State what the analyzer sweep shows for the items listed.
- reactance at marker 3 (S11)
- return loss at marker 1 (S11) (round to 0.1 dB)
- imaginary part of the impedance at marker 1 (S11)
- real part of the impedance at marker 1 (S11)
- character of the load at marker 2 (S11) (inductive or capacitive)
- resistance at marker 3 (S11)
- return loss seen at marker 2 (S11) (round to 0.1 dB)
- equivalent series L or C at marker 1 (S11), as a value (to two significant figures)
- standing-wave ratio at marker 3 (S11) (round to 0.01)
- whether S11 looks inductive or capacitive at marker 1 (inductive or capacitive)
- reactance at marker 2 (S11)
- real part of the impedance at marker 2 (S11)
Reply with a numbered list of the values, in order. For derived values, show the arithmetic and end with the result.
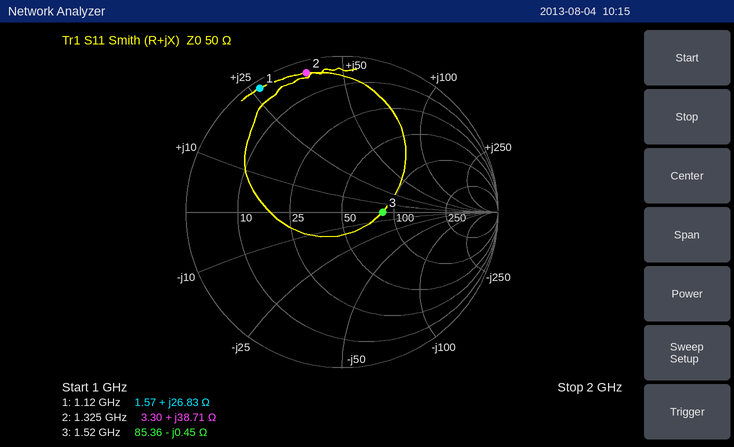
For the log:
1. -0.45 Ω
2. 0.4 dB
3. +26.83 Ω
4. 1.57 Ω
5. inductive
6. 85.36 Ω
7. 0.7 dB
8. L = 26.83 Ω/(2π × 1.12 GHz) ≈ 3.8 nH
9. 1.71
10. inductive
11. +38.71 Ω
12. 3.30 Ω
